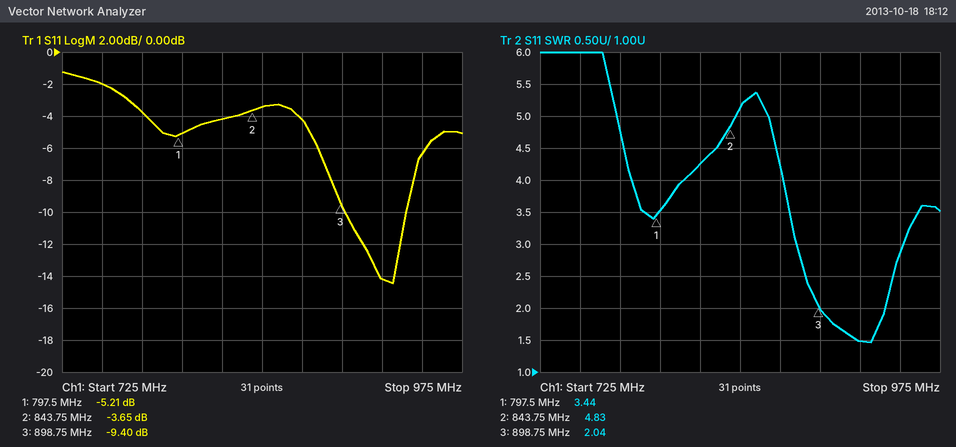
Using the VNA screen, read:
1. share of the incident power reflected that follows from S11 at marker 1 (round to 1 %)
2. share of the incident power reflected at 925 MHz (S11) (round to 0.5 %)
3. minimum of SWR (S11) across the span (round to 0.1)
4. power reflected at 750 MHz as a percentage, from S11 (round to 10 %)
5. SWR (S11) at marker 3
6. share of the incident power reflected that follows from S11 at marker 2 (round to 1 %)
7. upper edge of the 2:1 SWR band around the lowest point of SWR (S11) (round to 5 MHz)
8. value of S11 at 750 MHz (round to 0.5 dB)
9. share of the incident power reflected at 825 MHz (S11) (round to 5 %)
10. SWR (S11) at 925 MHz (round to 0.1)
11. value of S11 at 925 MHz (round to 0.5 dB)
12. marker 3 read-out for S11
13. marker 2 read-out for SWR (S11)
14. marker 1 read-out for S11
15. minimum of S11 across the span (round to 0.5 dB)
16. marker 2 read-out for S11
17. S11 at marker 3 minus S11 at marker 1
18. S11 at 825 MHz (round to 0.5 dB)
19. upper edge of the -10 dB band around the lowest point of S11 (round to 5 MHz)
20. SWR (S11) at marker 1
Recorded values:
30 %
4.0 %
1.5
60 %
2.04
43 %
940 MHz
-2.0 dB
40 %
1.5
-14.0 dB
-9.40 dB
4.83
-5.21 dB
-14.5 dB
-3.65 dB
-4.19 dB
-4.0 dB
940 MHz
3.44
